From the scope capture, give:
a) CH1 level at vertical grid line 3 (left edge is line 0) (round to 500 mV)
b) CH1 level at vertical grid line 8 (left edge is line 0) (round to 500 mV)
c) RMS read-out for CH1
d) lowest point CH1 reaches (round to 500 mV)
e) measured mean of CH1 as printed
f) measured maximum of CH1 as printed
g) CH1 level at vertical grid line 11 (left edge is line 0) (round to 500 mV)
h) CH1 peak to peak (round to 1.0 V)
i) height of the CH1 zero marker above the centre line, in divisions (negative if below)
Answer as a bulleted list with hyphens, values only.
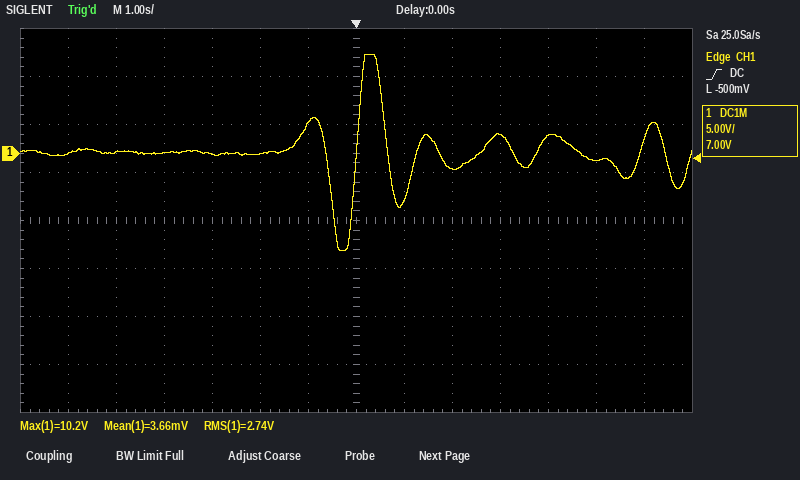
- 0.0 V
- -5.0 V
- 2.74 V
- -10.0 V
- 3.66 mV
- 10.2 V
- 2.0 V
- 20.0 V
- +1.4 div
